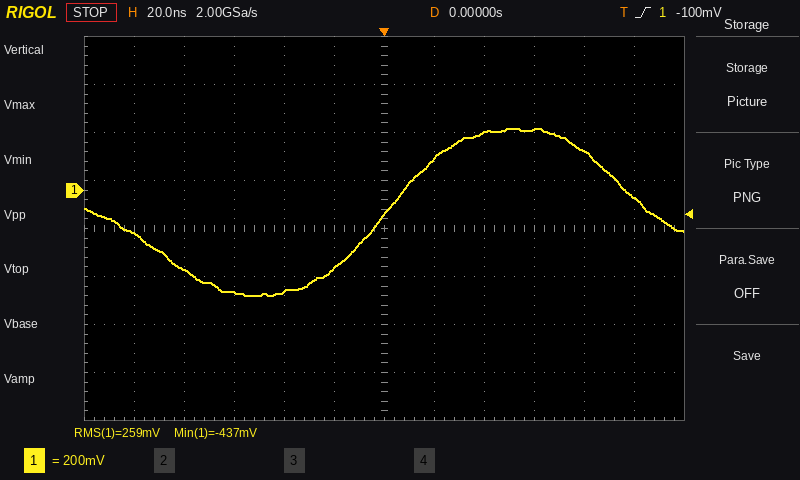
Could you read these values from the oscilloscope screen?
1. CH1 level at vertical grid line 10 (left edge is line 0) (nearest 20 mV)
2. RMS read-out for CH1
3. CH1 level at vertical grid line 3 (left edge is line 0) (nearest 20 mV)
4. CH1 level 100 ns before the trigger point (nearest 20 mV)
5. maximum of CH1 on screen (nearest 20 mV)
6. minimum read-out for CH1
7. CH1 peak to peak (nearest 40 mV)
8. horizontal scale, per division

160 mV
259 mV
-420 mV
-180 mV
260 mV
-437 mV
680 mV
20 ns
